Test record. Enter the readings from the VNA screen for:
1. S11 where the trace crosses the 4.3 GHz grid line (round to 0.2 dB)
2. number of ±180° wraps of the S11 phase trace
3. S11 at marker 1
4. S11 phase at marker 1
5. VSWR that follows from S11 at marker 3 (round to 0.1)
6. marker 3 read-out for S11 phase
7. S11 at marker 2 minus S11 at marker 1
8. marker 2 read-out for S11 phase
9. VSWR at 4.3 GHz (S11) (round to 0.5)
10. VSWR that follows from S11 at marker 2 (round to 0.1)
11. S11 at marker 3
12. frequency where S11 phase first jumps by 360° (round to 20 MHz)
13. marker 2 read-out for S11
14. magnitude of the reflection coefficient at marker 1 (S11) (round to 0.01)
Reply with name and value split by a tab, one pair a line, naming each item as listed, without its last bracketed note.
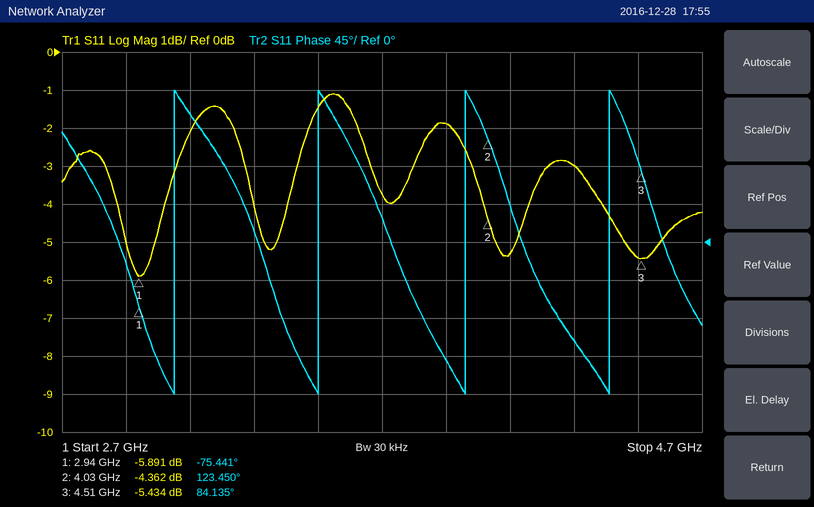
S11 where the trace crosses the 4.3 GHz grid line	-3.0 dB
number of ±180° wraps of the S11 phase trace	4
S11 at marker 1	-5.891 dB
S11 phase at marker 1	-75.441°
VSWR that follows from S11 at marker 3	3.3
marker 3 read-out for S11 phase	84.135°
S11 at marker 2 minus S11 at marker 1	1.529 dB
marker 2 read-out for S11 phase	123.450°
VSWR at 4.3 GHz (S11)	6.0
VSWR that follows from S11 at marker 2	4.1
S11 at marker 3	-5.434 dB
frequency where S11 phase first jumps by 360°	3.06 GHz
marker 2 read-out for S11	-4.362 dB
magnitude of the reflection coefficient at marker 1 (S11)	0.51
